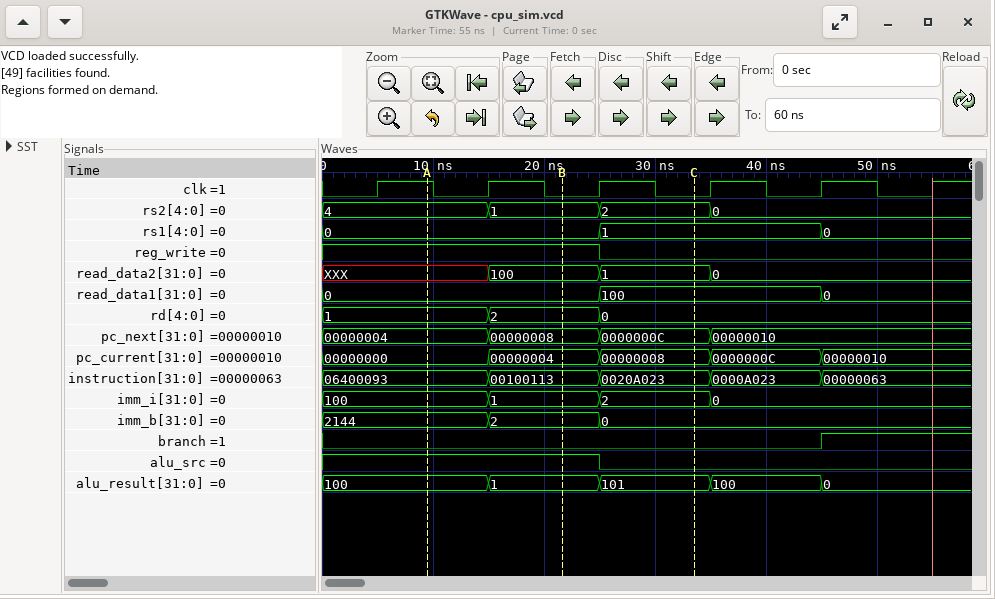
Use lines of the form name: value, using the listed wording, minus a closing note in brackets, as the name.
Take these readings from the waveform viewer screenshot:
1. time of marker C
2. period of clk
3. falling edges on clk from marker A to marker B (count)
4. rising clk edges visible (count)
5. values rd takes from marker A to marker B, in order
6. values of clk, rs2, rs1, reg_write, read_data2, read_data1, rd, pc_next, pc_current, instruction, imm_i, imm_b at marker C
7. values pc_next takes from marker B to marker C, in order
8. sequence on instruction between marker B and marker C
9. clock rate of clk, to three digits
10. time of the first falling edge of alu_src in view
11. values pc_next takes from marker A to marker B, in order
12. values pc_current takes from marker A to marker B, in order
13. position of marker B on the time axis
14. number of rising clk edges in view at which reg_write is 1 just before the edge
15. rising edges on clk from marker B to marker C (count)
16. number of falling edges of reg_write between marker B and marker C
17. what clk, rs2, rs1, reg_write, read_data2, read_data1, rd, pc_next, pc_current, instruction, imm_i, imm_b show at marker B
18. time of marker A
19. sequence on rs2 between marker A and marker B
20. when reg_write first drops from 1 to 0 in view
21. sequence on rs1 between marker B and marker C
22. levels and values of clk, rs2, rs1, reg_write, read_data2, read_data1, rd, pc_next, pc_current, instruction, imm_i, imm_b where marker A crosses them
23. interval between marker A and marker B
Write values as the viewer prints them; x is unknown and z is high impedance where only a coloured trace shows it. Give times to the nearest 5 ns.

time of marker C: 35 ns
period of clk: 10 ns
falling edges on clk from marker A to marker B: 2
rising clk edges visible: 6
values rd takes from marker A to marker B, in order: 1, 2
values of clk, rs2, rs1, reg_write, read_data2, read_data1, rd, pc_next, pc_current, instruction, imm_i, imm_b at marker C: clk=0, rs2=2, rs1=1, reg_write=0, read_data2=1, read_data1=100, rd=0, pc_next=0000000C, pc_current=00000008, instruction=0020A023, imm_i=2, imm_b=0
values pc_next takes from marker B to marker C, in order: 00000008, 0000000C
sequence on instruction between marker B and marker C: 00100113, 0020A023
clock rate of clk, to three digits: 100 MHz
time of the first falling edge of alu_src in view: 25 ns
values pc_next takes from marker A to marker B, in order: 00000004, 00000008
values pc_current takes from marker A to marker B, in order: 00000000, 00000004
position of marker B on the time axis: 20 ns
number of rising clk edges in view at which reg_write is 1 just before the edge: 3
rising edges on clk from marker B to marker C: 1
number of falling edges of reg_write between marker B and marker C: 1
what clk, rs2, rs1, reg_write, read_data2, read_data1, rd, pc_next, pc_current, instruction, imm_i, imm_b show at marker B: clk=0, rs2=1, rs1=0, reg_write=1, read_data2=100, read_data1=0, rd=2, pc_next=00000008, pc_current=00000004, instruction=00100113, imm_i=1, imm_b=2
time of marker A: 10 ns
sequence on rs2 between marker A and marker B: 4, 1
when reg_write first drops from 1 to 0 in view: 25 ns
sequence on rs1 between marker B and marker C: 0, 1
levels and values of clk, rs2, rs1, reg_write, read_data2, read_data1, rd, pc_next, pc_current, instruction, imm_i, imm_b where marker A crosses them: clk=1, rs2=4, rs1=0, reg_write=1, read_data2=XXX, read_data1=0, rd=1, pc_next=00000004, pc_current=00000000, instruction=06400093, imm_i=100, imm_b=2144
interval between marker A and marker B: 10 ns
